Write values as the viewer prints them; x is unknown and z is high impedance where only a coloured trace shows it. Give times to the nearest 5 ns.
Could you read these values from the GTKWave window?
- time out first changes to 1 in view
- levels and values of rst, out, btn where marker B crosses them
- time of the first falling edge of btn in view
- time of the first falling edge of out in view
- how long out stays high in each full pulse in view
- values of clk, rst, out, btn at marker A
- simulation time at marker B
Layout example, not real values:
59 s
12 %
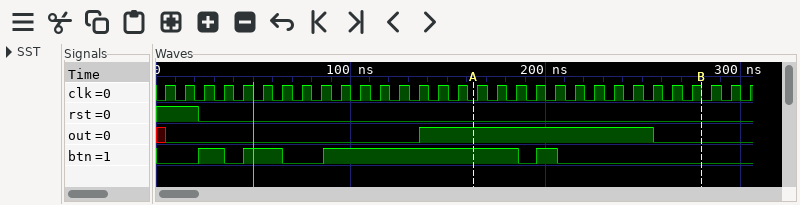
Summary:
135 ns
rst=0, out=0, btn=0
35 ns
255 ns
120 ns
clk=0, rst=0, out=1, btn=1
280 ns
